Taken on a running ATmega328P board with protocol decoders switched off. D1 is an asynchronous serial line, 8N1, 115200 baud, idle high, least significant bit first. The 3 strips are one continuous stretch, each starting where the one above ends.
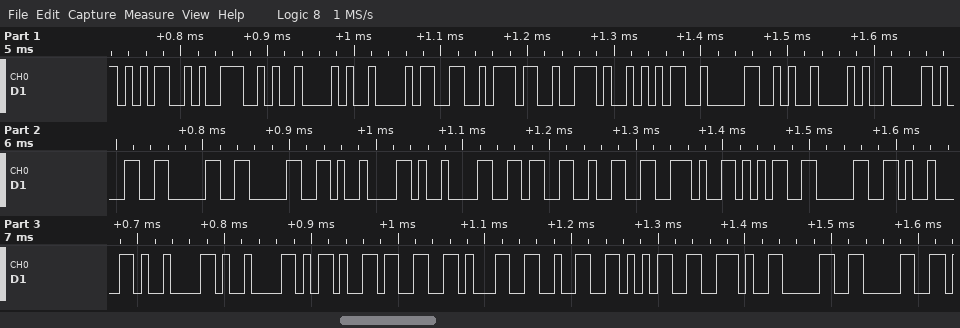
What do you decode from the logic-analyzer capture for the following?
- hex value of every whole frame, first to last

35 39 09 09 33 37 2E 35 30 09 09 31 30 30 09 09 36 32 2E 35 30 09 09 09 2D 33 31 32 35 2E 30 30
